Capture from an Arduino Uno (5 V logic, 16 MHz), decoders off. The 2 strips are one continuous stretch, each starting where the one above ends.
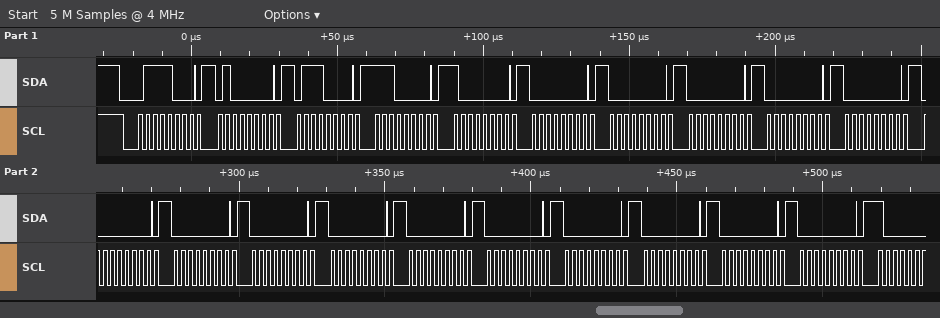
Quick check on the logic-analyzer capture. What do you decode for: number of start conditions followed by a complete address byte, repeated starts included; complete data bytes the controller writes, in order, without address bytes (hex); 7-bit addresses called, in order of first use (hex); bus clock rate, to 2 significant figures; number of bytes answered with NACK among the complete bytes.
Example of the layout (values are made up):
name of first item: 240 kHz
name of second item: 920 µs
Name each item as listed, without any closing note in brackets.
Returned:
number of start conditions followed by a complete address byte, repeated starts included: 1
complete data bytes the controller writes, in order, without address bytes: 40 70 E0 80 00 00 00 00 00 00 00 00 00 00 00 00 00 00 00
7-bit addresses called, in order of first use: 0x3C
bus clock rate, to 2 significant figures: 400 kHz
number of bytes answered with NACK among the complete bytes: 0
